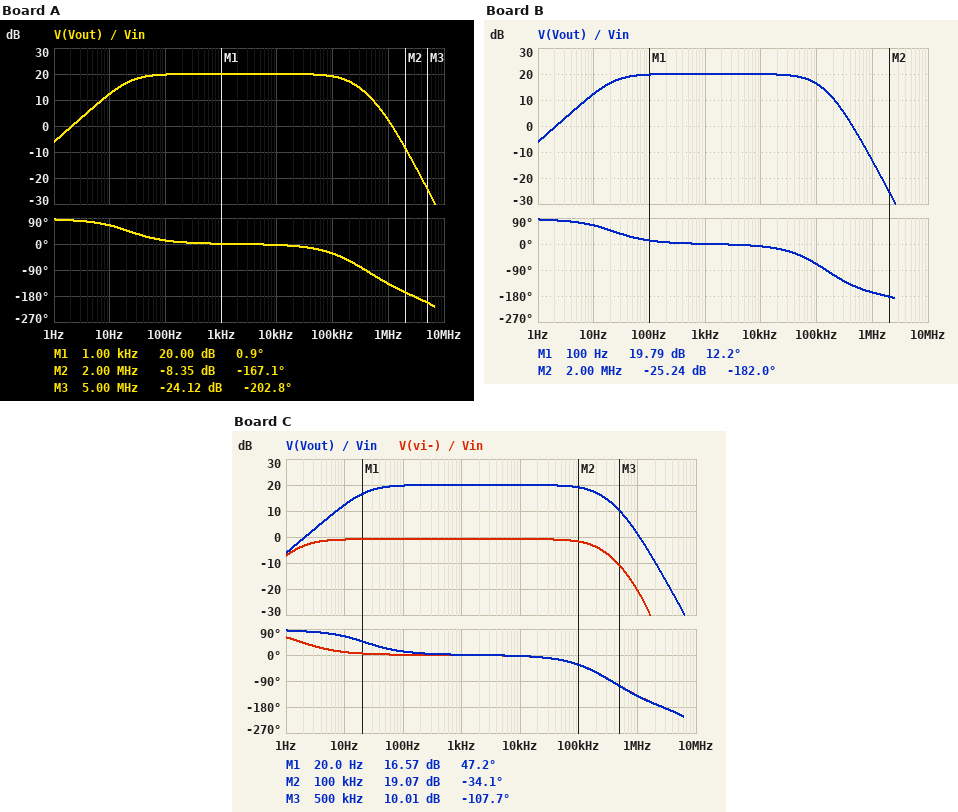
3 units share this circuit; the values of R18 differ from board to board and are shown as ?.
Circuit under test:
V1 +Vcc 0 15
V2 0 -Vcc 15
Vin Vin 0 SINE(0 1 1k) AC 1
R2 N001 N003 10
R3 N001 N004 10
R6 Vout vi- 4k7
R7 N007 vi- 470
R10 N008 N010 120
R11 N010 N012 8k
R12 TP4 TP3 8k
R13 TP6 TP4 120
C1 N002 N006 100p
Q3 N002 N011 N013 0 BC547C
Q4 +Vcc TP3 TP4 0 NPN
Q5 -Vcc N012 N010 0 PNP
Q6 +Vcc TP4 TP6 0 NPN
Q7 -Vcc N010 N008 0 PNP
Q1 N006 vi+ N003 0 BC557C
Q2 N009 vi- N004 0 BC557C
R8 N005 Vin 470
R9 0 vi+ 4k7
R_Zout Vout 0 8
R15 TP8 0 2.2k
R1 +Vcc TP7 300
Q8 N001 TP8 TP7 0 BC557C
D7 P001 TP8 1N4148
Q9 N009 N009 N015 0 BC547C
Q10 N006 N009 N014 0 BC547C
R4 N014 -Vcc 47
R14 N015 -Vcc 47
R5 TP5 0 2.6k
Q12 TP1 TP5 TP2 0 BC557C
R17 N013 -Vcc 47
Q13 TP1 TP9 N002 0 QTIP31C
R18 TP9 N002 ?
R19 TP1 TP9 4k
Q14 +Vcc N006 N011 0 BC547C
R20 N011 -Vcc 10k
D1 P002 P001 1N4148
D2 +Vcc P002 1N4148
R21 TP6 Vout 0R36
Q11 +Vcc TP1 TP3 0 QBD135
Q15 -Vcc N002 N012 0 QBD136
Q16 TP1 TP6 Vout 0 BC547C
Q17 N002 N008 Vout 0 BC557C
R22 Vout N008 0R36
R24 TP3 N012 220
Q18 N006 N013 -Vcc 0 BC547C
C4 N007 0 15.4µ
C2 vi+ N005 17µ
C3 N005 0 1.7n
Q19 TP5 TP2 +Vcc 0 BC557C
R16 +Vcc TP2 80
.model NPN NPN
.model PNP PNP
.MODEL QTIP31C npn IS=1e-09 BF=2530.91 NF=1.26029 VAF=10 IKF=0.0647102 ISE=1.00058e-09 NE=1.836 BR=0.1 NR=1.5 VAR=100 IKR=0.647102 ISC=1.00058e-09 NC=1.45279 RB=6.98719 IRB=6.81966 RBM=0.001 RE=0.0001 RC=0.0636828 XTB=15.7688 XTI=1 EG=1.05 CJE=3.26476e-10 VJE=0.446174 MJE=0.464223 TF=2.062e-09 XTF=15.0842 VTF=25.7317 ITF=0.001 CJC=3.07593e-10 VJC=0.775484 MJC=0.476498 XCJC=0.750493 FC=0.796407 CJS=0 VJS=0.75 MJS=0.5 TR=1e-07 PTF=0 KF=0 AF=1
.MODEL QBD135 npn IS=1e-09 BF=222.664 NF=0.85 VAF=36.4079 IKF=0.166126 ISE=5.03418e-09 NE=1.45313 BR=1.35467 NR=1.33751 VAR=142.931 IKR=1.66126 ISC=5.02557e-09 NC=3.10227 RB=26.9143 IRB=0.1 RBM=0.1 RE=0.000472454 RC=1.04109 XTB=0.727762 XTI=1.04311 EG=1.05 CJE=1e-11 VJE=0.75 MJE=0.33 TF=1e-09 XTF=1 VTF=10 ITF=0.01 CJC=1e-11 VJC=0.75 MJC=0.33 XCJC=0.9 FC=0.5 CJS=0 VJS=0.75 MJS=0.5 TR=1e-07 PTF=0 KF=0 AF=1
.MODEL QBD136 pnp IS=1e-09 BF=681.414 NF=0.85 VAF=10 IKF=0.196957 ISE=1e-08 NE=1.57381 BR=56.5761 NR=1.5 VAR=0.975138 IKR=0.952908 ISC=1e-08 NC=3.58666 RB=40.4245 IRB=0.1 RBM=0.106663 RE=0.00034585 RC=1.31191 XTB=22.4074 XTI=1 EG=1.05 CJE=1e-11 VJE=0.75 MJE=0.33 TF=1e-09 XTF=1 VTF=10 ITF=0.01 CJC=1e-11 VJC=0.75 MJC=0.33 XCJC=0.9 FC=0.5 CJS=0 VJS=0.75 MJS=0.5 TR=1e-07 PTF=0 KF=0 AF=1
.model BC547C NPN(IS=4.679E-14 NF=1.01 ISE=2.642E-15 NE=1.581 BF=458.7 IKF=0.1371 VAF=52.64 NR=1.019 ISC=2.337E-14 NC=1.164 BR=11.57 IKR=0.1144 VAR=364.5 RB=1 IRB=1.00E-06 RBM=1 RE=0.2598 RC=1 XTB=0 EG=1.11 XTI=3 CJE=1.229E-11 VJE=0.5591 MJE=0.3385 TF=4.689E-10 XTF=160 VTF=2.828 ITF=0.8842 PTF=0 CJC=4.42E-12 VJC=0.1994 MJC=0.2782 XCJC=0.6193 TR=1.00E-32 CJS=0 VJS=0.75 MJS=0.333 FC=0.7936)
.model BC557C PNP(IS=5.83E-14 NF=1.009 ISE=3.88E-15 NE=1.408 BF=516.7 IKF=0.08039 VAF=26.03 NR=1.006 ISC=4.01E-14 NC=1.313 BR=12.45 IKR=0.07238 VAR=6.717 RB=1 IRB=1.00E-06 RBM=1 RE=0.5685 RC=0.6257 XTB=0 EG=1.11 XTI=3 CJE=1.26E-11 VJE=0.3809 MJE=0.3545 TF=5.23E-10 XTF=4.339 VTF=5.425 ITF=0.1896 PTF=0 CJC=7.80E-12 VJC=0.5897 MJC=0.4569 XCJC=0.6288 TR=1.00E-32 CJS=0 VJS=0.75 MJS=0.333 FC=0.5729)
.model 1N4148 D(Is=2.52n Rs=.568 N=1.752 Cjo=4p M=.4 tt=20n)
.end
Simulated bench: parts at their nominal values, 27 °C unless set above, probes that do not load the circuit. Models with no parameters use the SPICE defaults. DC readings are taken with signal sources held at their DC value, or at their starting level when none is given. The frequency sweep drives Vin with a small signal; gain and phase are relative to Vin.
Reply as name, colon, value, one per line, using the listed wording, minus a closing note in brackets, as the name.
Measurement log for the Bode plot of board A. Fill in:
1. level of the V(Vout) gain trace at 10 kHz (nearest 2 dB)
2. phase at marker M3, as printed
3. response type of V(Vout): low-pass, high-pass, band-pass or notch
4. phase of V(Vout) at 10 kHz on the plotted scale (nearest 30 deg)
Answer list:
level of the V(Vout) gain trace at 10 kHz: 20 dB
phase at marker M3, as printed: -202.8 deg
response type of V(Vout): low-pass, high-pass, band-pass or notch: band-pass
phase of V(Vout) at 10 kHz on the plotted scale: 0 deg
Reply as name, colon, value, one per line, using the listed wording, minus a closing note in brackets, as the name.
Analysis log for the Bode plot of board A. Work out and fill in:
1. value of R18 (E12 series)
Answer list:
value of R18: 820 Ω
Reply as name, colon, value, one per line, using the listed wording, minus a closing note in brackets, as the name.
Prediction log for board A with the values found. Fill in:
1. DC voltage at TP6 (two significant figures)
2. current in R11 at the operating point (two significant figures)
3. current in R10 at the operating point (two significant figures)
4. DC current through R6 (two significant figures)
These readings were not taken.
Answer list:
DC voltage at TP6: 2.3 mV
current in R11 at the operating point: 100 µA
current in R10 at the operating point: 3.7 mA
DC current through R6: 3.2 µA
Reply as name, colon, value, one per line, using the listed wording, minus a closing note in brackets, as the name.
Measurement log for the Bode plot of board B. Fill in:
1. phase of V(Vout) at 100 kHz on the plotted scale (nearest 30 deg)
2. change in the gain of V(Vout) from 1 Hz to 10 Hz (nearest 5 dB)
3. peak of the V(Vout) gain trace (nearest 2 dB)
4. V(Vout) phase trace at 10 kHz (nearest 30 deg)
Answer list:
phase of V(Vout) at 100 kHz on the plotted scale: -60 deg
change in the gain of V(Vout) from 1 Hz to 10 Hz: 20 dB
peak of the V(Vout) gain trace: 20 dB
V(Vout) phase trace at 10 kHz: 0 deg
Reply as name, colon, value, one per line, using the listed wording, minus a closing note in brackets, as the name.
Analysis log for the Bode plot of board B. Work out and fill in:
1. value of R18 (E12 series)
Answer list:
value of R18: 2.2 kΩ
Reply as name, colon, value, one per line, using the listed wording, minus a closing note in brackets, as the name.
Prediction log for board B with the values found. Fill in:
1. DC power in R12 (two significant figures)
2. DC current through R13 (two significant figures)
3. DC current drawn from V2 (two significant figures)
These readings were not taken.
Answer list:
DC power in R12: 62 µW
DC current through R13: 150 µA
DC current drawn from V2: 18 mA
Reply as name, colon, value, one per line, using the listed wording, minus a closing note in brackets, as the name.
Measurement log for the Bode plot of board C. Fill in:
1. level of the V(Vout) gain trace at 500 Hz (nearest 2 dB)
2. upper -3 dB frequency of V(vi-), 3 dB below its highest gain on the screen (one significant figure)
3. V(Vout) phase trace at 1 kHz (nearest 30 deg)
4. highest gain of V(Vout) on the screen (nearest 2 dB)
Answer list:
level of the V(Vout) gain trace at 500 Hz: 20 dB
upper -3 dB frequency of V(vi-), 3 dB below its highest gain on the screen: 200 kHz
V(Vout) phase trace at 1 kHz: 0 deg
highest gain of V(Vout) on the screen: 20 dB
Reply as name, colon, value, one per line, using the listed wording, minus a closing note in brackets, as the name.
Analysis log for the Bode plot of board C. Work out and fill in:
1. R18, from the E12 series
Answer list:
R18, from the E12 series: 1.2 kΩ
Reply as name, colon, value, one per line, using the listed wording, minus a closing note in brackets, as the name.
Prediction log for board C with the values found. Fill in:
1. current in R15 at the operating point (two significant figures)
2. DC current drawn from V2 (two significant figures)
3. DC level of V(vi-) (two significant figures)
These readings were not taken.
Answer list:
current in R15 at the operating point: 5.9 mA
DC current drawn from V2: 22 mA
DC level of V(vi-): 16 mV
